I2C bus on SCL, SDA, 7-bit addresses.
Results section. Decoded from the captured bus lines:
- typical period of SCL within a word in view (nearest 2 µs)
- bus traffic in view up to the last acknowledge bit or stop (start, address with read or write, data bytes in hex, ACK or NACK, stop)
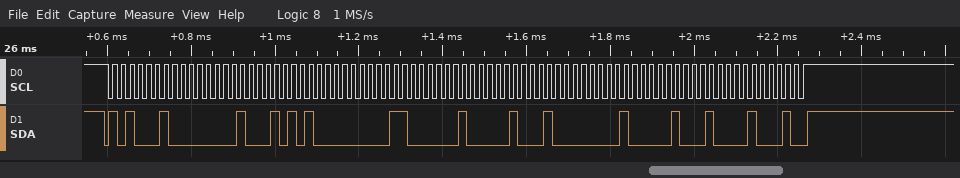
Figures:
20 µs
start, address 51 write ACK, 02 ACK, 54 ACK, 03 ACK, 04 ACK, 22 ACK, 02 ACK, 11 ACK, 11 ACK, stop
